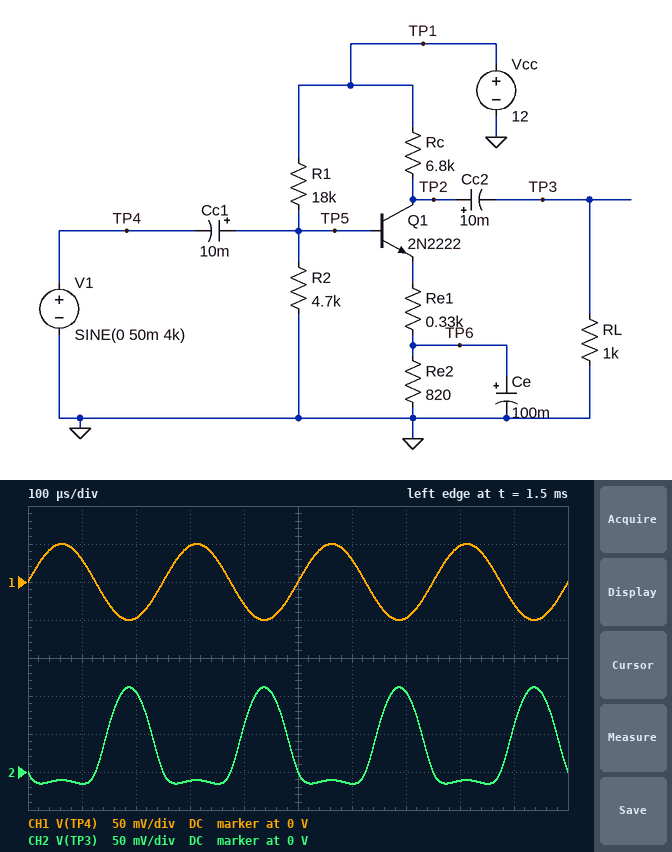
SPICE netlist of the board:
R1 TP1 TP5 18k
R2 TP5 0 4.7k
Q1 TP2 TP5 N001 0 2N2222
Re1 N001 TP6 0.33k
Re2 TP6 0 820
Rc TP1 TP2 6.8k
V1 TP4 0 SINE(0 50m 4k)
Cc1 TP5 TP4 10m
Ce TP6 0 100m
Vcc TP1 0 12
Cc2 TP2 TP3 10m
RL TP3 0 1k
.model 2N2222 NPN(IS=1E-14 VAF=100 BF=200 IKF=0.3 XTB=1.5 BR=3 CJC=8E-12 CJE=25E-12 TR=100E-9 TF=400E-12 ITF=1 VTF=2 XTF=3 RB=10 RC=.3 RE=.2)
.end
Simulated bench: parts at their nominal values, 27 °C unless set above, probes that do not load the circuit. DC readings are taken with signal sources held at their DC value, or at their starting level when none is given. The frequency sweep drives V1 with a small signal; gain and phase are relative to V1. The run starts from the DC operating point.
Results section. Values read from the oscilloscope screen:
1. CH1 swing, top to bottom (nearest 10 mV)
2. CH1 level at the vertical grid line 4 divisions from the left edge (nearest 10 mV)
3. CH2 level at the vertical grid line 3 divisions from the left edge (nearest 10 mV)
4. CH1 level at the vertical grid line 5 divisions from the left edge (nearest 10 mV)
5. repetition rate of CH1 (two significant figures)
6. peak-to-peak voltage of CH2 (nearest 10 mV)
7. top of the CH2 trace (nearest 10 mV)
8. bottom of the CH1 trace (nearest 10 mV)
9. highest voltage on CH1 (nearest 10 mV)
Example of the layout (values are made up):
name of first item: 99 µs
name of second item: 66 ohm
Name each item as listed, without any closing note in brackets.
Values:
CH1 swing, top to bottom: 100 mV
CH1 level at the vertical grid line 4 divisions from the left edge: -30 mV
CH2 level at the vertical grid line 3 divisions from the left edge: -10 mV
CH1 level at the vertical grid line 5 divisions from the left edge: 0 V
repetition rate of CH1: 4.0 kHz
peak-to-peak voltage of CH2: 130 mV
top of the CH2 trace: 110 mV
bottom of the CH1 trace: -50 mV
highest voltage on CH1: 50 mV
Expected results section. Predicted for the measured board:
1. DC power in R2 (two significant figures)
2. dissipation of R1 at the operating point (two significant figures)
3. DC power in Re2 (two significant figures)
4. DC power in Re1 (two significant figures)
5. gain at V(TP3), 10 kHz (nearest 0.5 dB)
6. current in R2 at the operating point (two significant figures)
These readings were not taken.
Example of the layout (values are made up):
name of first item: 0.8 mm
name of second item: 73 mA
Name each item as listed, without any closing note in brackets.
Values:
DC power in R2: 1.2 mW
dissipation of R1 at the operating point: 5.1 mW
DC power in Re2: 1.9 mW
DC power in Re1: 760 µW
gain at V(TP3), 10 kHz: 2.5 dB
current in R2 at the operating point: 510 µA
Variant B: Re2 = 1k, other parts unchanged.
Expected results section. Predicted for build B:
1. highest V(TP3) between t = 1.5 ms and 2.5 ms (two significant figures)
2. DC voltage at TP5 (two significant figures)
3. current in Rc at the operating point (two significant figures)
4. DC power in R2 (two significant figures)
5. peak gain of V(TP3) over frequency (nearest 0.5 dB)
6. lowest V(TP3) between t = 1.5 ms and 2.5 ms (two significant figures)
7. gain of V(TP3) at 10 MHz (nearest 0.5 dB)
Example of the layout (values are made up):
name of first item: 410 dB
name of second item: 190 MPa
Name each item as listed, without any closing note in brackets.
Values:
highest V(TP3) between t = 1.5 ms and 2.5 ms: 120 mV
DC voltage at TP5: 2.5 V
current in Rc at the operating point: 1.3 mA
DC power in R2: 1.3 mW
peak gain of V(TP3) over frequency: 8.0 dB
lowest V(TP3) between t = 1.5 ms and 2.5 ms: -120 mV
gain of V(TP3) at 10 MHz: 7.5 dB
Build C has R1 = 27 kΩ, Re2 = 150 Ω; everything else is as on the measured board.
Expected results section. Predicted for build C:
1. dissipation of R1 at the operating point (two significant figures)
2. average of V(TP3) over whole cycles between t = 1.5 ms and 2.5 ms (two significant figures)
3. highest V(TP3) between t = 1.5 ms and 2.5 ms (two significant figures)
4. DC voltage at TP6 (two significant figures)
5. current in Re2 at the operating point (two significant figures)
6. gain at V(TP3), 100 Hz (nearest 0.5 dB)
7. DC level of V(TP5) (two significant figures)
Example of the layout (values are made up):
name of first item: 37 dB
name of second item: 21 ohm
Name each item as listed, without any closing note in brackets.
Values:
dissipation of R1 at the operating point: 4.1 mW
average of V(TP3) over whole cycles between t = 1.5 ms and 2.5 ms: 20 mV
highest V(TP3) between t = 1.5 ms and 2.5 ms: 63 mV
DC voltage at TP6: 260 mV
current in Re2 at the operating point: 1.7 mA
gain at V(TP3), 100 Hz: -27.5 dB
DC level of V(TP5): 1.5 V
